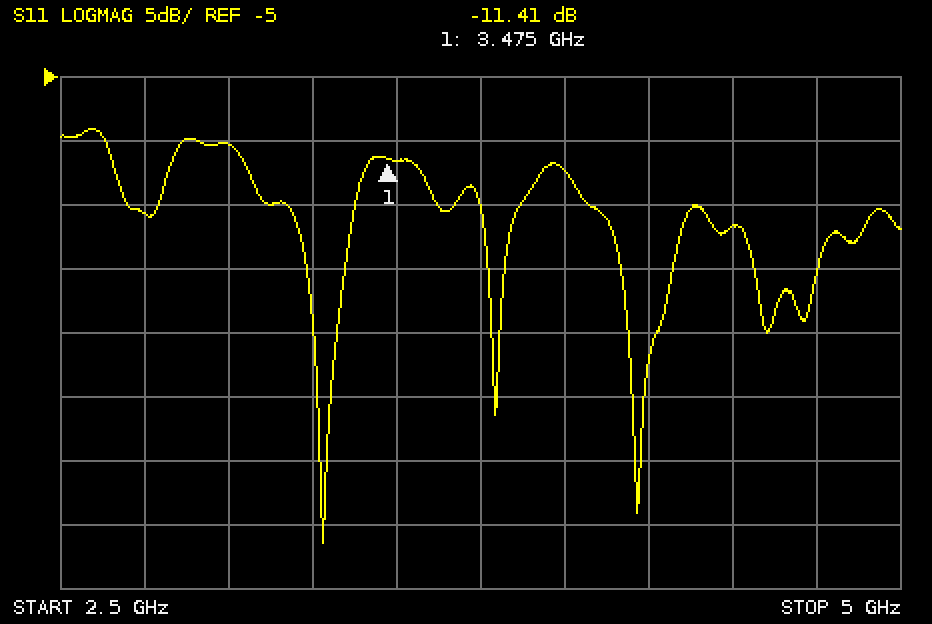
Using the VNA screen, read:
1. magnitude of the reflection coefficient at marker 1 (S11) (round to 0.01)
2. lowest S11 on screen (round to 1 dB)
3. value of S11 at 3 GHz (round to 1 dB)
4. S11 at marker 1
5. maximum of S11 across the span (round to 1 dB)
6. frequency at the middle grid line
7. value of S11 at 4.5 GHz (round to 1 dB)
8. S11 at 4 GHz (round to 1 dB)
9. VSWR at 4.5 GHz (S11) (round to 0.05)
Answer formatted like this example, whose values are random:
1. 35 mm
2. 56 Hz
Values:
1. 0.27
2. -41 dB
3. -10 dB
4. -11.41 dB
5. -9 dB
6. 3.75 GHz
7. -17 dB
8. -12 dB
9. 1.35
